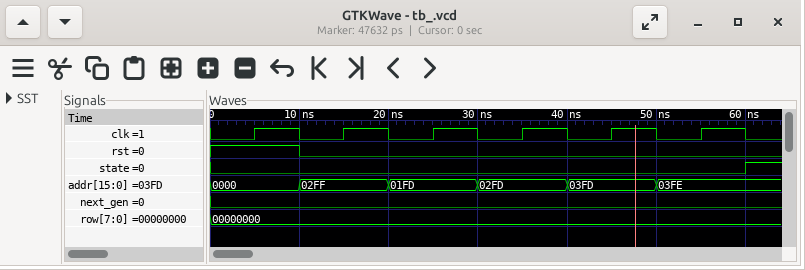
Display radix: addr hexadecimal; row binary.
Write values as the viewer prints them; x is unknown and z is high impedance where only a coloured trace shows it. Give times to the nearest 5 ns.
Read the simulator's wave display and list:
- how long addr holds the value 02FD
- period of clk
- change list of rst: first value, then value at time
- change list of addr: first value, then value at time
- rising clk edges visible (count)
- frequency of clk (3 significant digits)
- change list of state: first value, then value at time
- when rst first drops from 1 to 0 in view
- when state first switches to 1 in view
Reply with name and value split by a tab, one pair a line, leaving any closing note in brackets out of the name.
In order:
how long addr holds the value 02FD	10 ns
period of clk	10 ns
change list of rst: first value, then value at time	1, 0 at 10 ns
change list of addr: first value, then value at time	0000, 02FF at 10 ns, 01FD at 20 ns, 02FD at 30 ns, 03FD at 40 ns, 03FE at 50 ns
rising clk edges visible	6
frequency of clk	100 MHz
change list of state: first value, then value at time	0, 1 at 60 ns
when rst first drops from 1 to 0 in view	10 ns
when state first switches to 1 in view	60 ns
